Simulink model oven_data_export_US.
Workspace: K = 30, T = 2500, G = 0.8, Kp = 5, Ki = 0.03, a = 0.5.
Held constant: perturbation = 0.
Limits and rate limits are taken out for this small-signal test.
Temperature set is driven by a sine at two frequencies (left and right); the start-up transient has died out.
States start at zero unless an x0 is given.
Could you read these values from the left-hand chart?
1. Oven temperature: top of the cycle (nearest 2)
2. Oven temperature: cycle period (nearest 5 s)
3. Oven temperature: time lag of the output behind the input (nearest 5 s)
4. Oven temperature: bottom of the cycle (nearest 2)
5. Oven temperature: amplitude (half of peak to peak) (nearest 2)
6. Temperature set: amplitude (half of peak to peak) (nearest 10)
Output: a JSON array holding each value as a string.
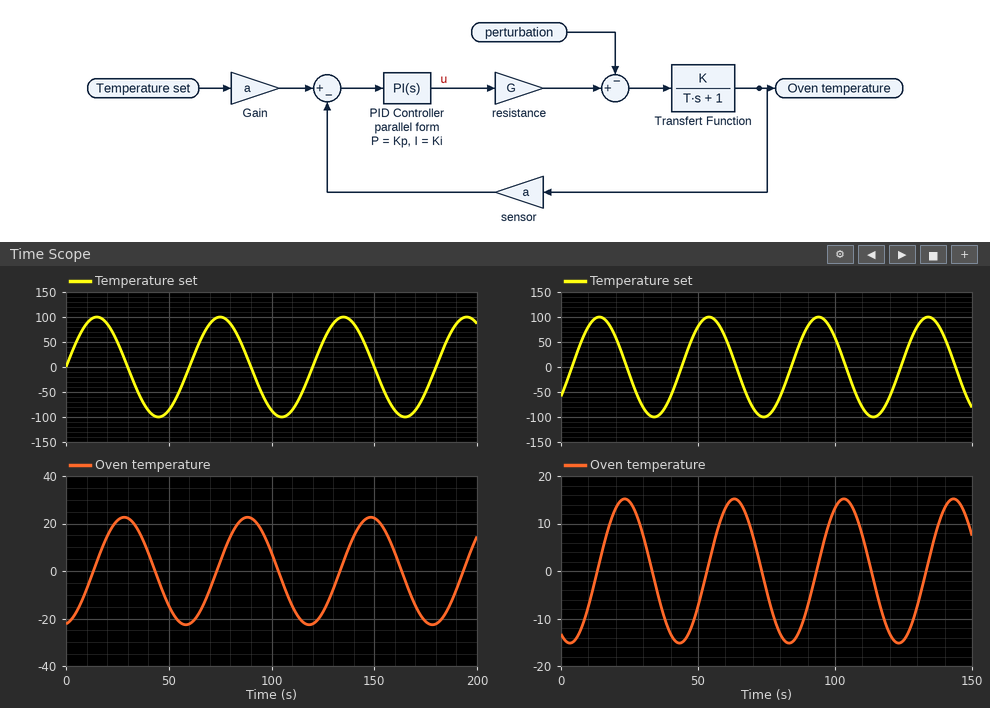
["22", "60 s", "15 s", "-22", "22", "100"]
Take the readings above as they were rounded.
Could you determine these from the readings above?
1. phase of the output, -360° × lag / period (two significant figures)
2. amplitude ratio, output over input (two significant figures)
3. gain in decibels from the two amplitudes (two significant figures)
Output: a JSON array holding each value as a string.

["-90°", "0.22", "-13 dB"]
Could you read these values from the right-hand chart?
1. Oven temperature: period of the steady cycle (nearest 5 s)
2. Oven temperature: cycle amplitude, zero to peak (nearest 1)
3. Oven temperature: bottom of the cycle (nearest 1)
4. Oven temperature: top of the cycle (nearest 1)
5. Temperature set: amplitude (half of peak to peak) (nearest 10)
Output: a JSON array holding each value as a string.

["40 s", "15", "-15", "15", "100"]
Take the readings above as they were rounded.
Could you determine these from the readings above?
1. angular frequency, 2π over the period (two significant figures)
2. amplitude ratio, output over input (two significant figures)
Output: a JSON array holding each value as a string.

["0.16 rad/s", "0.15"]
